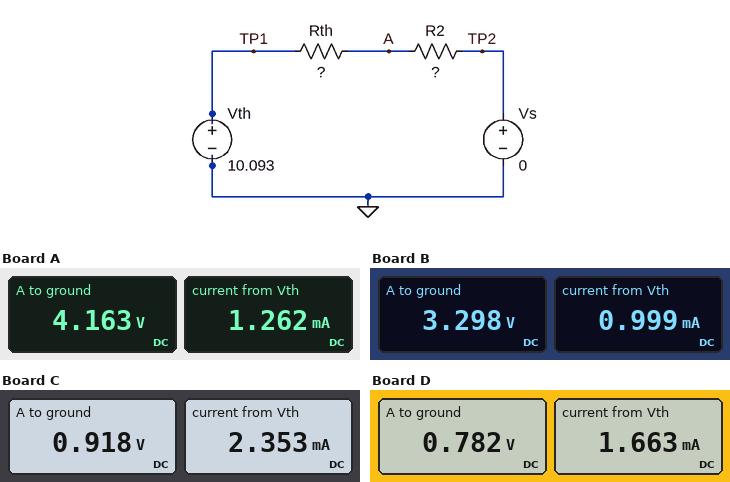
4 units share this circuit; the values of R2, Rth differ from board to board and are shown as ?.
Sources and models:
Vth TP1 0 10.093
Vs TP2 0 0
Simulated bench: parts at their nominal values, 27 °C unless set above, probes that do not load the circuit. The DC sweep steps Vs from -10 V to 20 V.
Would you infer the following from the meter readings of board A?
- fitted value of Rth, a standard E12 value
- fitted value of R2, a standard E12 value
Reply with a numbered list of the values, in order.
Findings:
1. 4.7 kΩ
2. 3.3 kΩ
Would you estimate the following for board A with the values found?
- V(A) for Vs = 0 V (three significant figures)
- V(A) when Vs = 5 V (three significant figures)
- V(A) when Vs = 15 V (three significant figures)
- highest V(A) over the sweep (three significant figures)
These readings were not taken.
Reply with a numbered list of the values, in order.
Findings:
1. 4.16 V
2. 7.10 V
3. 13.0 V
4. 15.9 V
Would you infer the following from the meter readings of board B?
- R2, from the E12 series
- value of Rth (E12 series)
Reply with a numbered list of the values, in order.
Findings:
1. 3.3 kΩ
2. 6.8 kΩ
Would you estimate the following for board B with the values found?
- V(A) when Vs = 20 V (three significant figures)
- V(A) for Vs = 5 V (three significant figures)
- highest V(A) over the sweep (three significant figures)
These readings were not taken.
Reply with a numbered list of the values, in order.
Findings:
1. 16.8 V
2. 6.66 V
3. 16.8 V
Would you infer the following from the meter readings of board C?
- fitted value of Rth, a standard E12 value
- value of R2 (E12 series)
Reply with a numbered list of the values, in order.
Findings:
1. 3.9 kΩ
2. 390 Ω
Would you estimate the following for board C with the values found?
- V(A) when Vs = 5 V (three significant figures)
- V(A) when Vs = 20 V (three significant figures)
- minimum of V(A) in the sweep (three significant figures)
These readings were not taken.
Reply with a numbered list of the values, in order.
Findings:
1. 5.46 V
2. 19.1 V
3. -8.17 V
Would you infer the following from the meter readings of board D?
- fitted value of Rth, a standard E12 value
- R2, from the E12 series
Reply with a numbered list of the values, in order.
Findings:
1. 5.6 kΩ
2. 470 Ω
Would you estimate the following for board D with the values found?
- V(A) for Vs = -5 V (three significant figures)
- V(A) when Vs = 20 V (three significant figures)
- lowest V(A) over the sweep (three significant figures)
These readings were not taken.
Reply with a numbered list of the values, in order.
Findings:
1. -3.83 V
2. 19.2 V
3. -8.44 V
